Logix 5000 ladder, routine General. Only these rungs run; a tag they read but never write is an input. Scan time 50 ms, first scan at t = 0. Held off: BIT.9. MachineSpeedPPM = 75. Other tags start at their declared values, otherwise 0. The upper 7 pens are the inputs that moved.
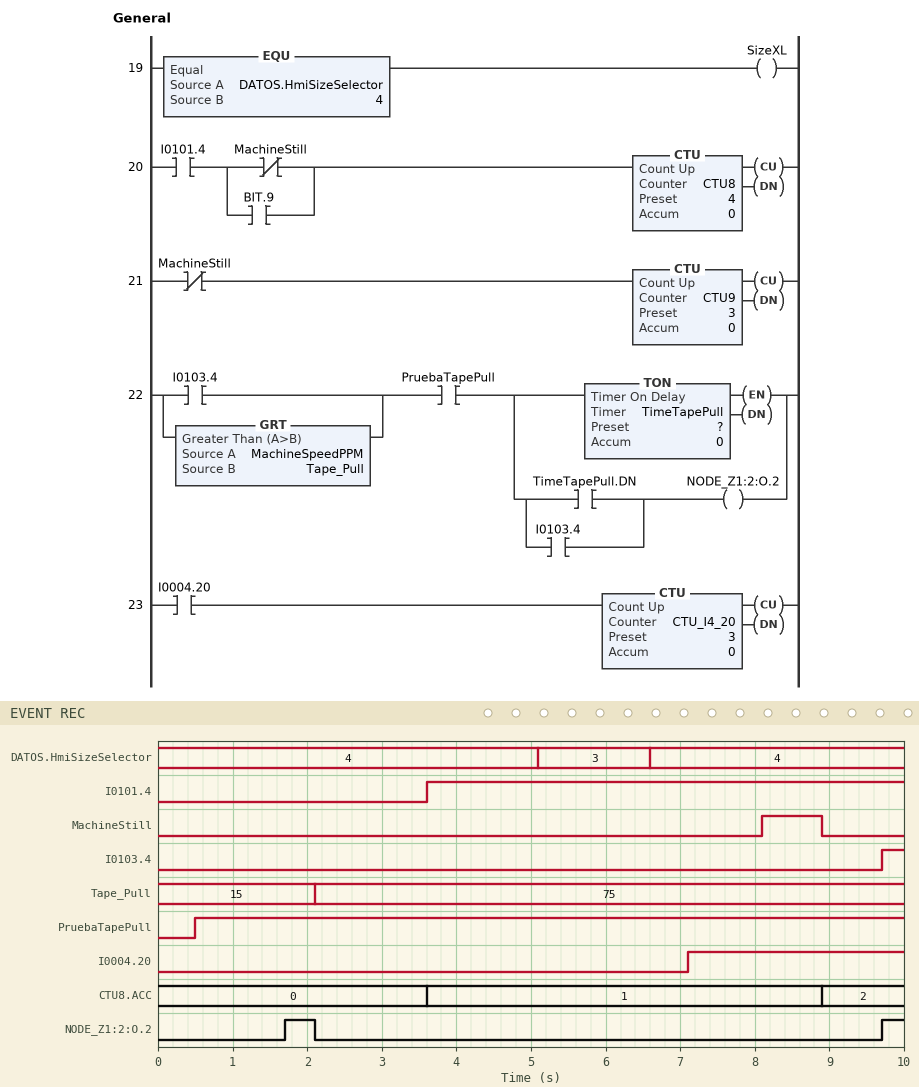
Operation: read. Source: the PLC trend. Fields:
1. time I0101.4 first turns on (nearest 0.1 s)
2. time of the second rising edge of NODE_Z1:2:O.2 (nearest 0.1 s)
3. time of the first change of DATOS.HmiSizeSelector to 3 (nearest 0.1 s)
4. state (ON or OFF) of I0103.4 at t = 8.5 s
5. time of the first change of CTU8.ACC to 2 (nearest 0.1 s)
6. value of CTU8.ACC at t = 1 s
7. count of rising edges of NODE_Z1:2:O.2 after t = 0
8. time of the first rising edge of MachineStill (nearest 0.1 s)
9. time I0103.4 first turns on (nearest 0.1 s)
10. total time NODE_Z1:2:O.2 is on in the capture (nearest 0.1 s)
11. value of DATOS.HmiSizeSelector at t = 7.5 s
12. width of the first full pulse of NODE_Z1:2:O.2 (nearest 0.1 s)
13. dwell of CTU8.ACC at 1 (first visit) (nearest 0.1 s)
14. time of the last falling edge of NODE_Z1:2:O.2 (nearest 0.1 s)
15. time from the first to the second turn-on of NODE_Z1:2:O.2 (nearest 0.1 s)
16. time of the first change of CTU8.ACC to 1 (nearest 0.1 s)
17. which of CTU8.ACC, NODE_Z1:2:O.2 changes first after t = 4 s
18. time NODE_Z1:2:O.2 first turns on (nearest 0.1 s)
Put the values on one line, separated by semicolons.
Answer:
3.6 s; 9.7 s; 5.1 s; OFF; 8.9 s; 0; 2; 8.1 s; 9.7 s; 0.7 s; 4; 0.4 s; 5.3 s; 2.1 s; 8.0 s; 3.6 s; CTU8.ACC; 1.7 s
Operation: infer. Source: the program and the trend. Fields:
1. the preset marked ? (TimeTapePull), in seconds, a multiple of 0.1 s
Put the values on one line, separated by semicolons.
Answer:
1.2 s
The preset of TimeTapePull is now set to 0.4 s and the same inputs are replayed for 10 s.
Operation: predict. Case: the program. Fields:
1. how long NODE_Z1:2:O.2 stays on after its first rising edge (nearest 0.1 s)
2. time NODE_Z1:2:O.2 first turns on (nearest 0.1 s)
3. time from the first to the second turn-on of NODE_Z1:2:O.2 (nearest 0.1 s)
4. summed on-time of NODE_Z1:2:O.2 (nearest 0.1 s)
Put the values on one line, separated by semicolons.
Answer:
1.2 s; 0.9 s; 8.8 s; 1.5 s
